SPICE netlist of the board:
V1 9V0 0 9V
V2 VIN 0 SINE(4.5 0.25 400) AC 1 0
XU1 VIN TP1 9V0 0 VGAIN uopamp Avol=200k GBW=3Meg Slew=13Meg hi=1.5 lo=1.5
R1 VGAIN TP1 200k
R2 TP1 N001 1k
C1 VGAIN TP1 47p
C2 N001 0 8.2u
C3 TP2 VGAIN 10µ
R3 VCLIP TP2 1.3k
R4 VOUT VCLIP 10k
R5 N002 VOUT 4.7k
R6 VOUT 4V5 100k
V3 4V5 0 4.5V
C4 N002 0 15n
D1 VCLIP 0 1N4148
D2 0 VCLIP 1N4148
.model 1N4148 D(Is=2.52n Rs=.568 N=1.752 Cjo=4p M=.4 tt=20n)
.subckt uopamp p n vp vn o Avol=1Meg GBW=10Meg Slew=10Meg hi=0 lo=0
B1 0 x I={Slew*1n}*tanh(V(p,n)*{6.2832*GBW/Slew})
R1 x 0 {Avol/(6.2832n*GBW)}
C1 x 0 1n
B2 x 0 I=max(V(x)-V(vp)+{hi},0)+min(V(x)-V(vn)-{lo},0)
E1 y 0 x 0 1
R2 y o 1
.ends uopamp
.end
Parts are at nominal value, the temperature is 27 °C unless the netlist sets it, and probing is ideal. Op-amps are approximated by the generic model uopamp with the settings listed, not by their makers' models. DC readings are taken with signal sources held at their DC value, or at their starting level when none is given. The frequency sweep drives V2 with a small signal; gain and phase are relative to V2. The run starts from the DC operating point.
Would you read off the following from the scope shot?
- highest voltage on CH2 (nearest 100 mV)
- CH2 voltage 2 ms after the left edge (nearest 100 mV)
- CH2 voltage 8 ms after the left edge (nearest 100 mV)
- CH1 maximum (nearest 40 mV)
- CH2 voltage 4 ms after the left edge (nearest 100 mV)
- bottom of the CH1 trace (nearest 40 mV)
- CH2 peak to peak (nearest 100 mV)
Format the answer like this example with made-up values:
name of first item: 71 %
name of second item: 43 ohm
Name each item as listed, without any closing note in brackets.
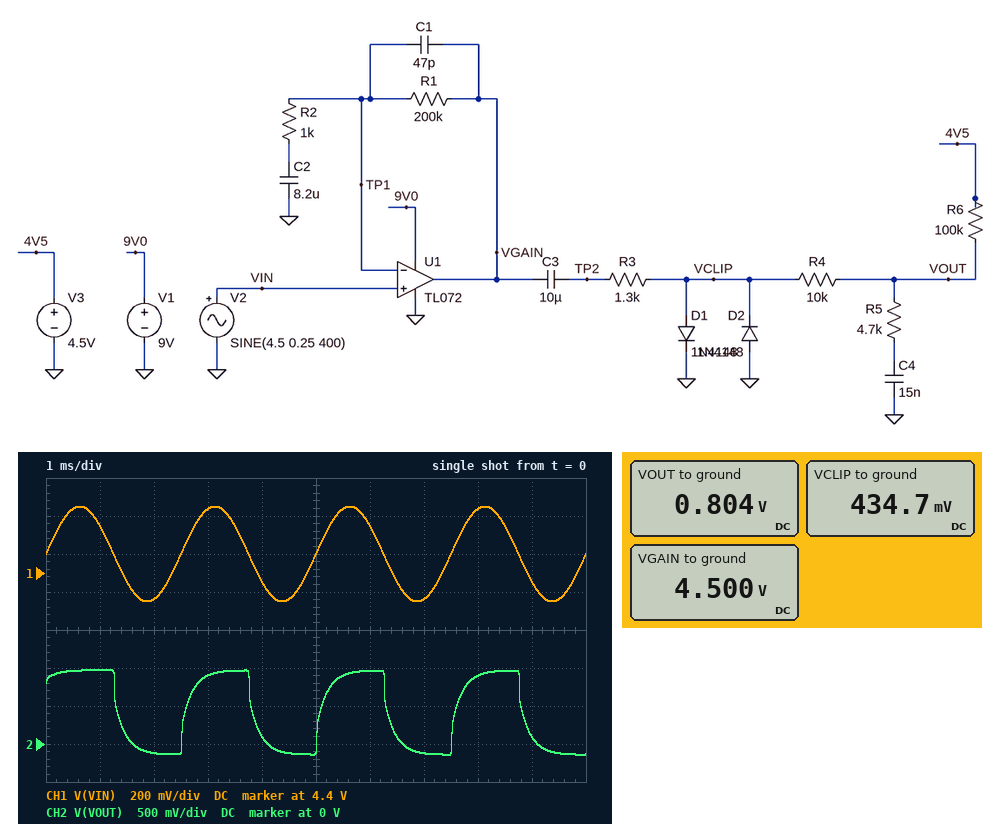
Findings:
highest voltage on CH2: 1.0 V
CH2 voltage 2 ms after the left edge: -100 mV
CH2 voltage 8 ms after the left edge: 900 mV
CH1 maximum: 4.76 V
CH2 voltage 4 ms after the left edge: 100 mV
bottom of the CH1 trace: 4.24 V
CH2 peak to peak: 1.1 V
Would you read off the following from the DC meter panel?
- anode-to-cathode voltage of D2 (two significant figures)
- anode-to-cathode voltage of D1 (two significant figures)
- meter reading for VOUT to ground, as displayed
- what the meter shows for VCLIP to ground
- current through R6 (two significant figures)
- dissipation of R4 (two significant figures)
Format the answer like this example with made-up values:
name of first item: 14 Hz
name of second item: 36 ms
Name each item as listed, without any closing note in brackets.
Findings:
anode-to-cathode voltage of D2: -430 mV
anode-to-cathode voltage of D1: 430 mV
meter reading for VOUT to ground, as displayed: 0.804 V
what the meter shows for VCLIP to ground: 434.7 mV
current through R6: 37 µA
dissipation of R4: 14 µW
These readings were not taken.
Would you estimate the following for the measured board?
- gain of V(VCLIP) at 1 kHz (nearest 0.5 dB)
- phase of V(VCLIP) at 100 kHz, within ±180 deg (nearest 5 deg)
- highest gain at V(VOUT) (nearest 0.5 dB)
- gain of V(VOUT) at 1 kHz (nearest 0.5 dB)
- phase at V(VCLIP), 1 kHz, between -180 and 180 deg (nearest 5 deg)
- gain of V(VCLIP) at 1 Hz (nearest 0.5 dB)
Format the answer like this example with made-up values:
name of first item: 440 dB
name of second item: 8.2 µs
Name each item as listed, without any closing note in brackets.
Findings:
gain of V(VCLIP) at 1 kHz: 39.5 dB
phase of V(VCLIP) at 100 kHz, within ±180 deg: -85 deg
highest gain at V(VOUT): 38.5 dB
gain of V(VOUT) at 1 kHz: 35.0 dB
phase at V(VCLIP), 1 kHz, between -180 and 180 deg: -5 deg
gain of V(VCLIP) at 1 Hz: -2.0 dB
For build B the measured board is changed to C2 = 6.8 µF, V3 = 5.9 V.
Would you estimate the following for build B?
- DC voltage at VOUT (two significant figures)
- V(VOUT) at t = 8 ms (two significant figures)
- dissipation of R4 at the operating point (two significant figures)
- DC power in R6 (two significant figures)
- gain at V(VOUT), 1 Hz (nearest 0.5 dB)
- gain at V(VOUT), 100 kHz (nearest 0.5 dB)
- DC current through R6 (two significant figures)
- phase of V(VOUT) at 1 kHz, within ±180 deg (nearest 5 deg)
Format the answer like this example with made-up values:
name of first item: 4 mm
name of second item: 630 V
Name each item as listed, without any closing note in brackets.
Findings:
DC voltage at VOUT: 940 mV
V(VOUT) at t = 8 ms: 1.0 V
dissipation of R4 at the operating point: 25 µW
DC power in R6: 250 µW
gain at V(VOUT), 1 Hz: -7.0 dB
gain at V(VOUT), 100 kHz: 6.0 dB
DC current through R6: 50 µA
phase of V(VOUT) at 1 kHz, within ±180 deg: -35 deg
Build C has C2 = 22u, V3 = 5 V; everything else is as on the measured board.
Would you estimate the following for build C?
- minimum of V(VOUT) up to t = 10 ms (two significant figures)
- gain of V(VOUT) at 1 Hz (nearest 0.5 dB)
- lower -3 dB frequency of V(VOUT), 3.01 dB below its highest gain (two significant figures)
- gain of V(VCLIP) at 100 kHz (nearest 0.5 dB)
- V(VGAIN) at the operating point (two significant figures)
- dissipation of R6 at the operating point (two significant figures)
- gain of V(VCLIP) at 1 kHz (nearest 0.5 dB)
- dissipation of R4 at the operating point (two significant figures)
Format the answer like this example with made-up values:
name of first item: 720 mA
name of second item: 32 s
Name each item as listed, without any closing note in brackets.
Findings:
minimum of V(VOUT) up to t = 10 ms: -95 mV
gain of V(VOUT) at 1 Hz: 4.5 dB
lower -3 dB frequency of V(VOUT), 3.01 dB below its highest gain: 11 Hz
gain of V(VCLIP) at 100 kHz: 17.0 dB
V(VGAIN) at the operating point: 4.5 V
dissipation of R6 at the operating point: 170 µW
gain of V(VCLIP) at 1 kHz: 39.0 dB
dissipation of R4 at the operating point: 17 µW
